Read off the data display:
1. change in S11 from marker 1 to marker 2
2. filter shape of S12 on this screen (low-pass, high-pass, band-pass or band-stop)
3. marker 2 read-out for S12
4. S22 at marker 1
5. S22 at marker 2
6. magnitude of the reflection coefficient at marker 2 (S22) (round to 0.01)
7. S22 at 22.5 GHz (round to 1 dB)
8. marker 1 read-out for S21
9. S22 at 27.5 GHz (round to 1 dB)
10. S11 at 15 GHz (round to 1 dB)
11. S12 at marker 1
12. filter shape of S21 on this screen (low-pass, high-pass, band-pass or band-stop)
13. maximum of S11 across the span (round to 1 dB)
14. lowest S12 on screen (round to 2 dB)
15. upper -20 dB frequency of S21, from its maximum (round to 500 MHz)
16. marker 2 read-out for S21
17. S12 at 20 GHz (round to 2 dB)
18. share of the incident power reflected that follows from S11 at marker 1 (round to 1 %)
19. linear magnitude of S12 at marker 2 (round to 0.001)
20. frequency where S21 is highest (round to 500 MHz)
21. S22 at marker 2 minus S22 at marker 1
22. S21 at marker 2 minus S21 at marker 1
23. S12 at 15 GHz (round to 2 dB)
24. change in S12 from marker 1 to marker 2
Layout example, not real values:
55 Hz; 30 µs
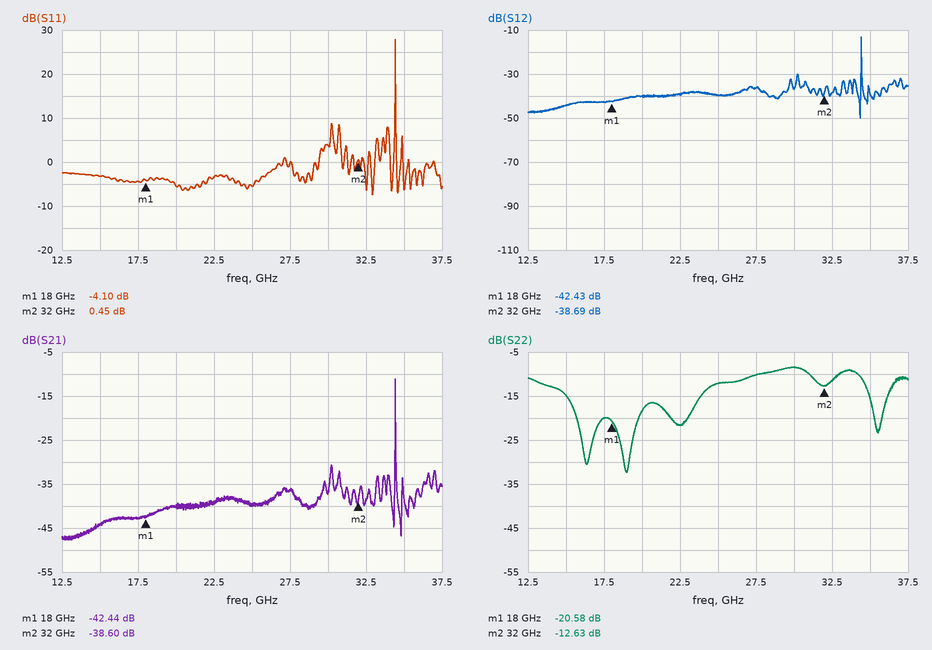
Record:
4.55 dB; band-pass; -38.69 dB; -20.58 dB; -12.63 dB; 0.23; -22 dB; -42.44 dB; -10 dB; -3 dB; -42.43 dB; band-pass; 28 dB; -50 dB; 34.5 GHz; -38.60 dB; -40 dB; 39 %; 0.012; 34.5 GHz; 7.95 dB; 3.84 dB; -44 dB; 3.74 dB
